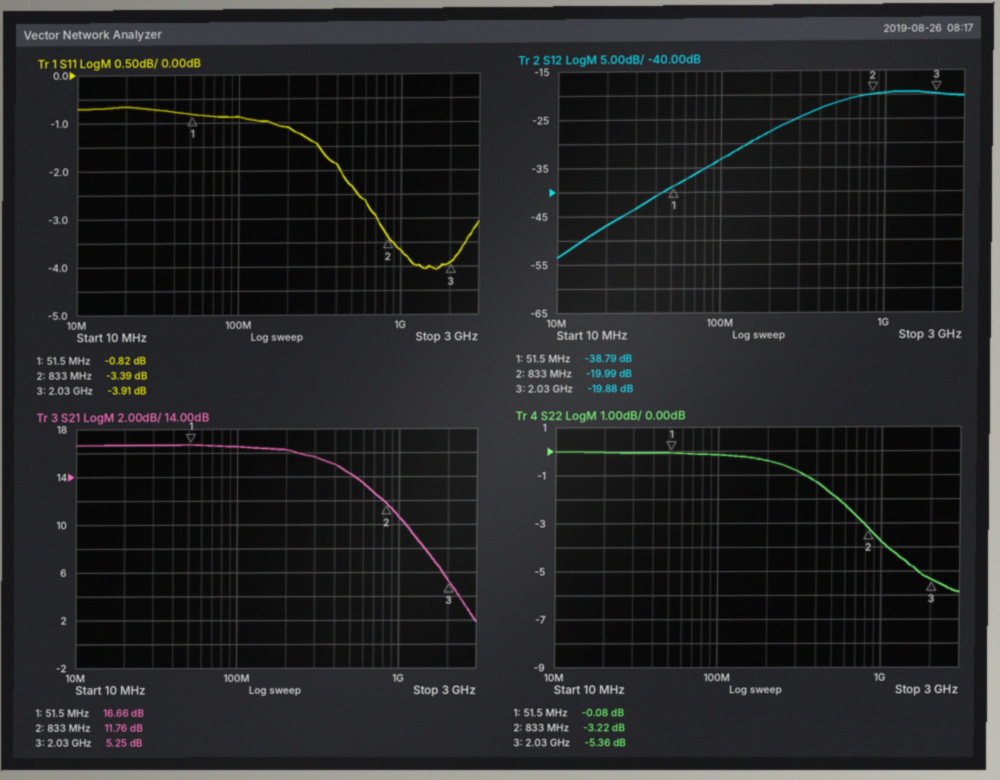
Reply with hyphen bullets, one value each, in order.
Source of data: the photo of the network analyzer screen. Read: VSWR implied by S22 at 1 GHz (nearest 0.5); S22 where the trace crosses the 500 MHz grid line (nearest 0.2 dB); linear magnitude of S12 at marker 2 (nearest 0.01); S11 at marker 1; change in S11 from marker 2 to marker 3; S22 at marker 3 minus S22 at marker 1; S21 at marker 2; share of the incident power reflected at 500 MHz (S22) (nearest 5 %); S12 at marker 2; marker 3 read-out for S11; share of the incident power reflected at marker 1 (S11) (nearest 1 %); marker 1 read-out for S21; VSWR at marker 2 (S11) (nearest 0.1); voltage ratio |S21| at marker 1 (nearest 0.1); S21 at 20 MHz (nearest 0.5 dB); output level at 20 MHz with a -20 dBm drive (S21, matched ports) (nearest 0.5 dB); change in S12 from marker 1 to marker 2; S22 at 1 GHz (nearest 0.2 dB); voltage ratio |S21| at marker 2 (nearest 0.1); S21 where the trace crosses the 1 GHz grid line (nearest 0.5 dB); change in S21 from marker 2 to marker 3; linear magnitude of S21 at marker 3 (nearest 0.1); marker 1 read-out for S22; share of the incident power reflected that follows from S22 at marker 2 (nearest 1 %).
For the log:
- 4.5
- -1.8 dB
- 0.10
- -0.82 dB
- -0.52 dB
- -5.28 dB
- 11.76 dB
- 65 %
- -19.99 dB
- -3.91 dB
- 83 %
- 16.66 dB
- 5.2
- 6.8
- 16.5 dB
- -3.5 dBm
- 18.80 dB
- -3.8 dB
- 3.9
- 10.5 dB
- -6.51 dB
- 1.8
- -0.08 dB
- 48 %
